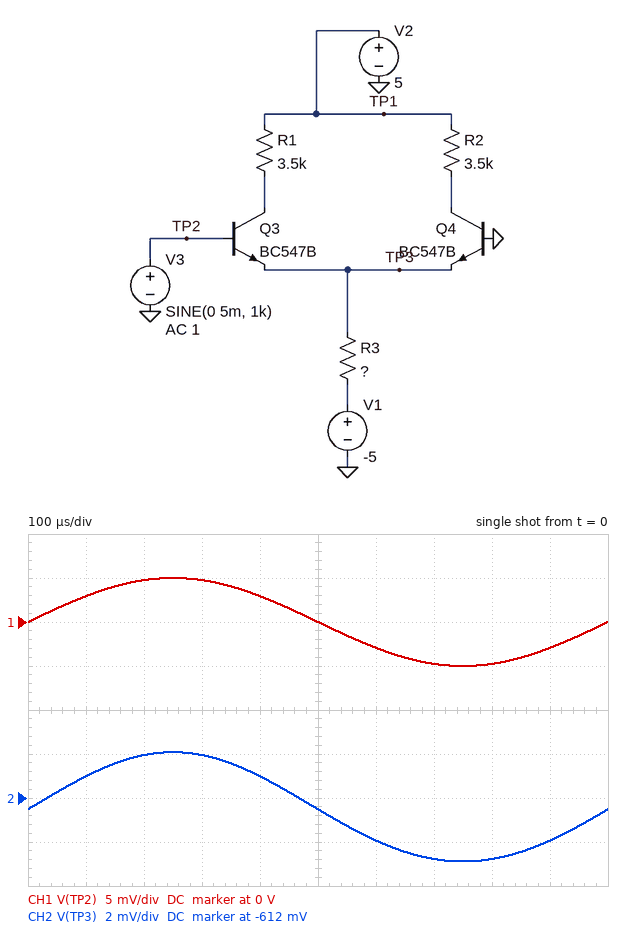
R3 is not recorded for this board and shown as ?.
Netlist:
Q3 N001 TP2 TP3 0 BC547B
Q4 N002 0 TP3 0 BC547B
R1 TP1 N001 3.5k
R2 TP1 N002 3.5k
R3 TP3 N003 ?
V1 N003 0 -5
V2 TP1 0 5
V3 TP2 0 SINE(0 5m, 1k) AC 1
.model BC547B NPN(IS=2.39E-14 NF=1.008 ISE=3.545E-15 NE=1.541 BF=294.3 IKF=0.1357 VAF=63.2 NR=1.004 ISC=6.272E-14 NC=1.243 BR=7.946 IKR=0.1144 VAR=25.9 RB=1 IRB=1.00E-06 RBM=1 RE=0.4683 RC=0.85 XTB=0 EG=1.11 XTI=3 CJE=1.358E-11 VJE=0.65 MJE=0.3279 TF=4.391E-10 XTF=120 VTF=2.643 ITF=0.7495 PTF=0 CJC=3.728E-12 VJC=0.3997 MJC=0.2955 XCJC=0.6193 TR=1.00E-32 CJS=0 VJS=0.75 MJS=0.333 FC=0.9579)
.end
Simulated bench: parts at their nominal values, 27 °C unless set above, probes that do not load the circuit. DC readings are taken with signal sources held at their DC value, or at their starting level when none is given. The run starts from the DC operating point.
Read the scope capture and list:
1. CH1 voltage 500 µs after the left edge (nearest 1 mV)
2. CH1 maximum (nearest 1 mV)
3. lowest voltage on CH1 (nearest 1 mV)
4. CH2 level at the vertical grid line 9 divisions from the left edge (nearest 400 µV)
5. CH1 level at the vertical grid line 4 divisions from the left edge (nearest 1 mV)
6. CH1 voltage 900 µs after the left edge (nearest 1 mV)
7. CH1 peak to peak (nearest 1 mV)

0 V
5 mV
-5 mV
-614.0 mV
3 mV
-3 mV
10 mV
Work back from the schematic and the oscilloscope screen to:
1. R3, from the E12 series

5.6 kΩ
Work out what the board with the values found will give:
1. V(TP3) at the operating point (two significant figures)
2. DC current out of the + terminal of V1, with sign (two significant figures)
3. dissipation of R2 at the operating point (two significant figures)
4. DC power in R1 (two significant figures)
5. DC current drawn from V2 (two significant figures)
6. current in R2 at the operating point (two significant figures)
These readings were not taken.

-610 mV
-780 µA
530 µW
530 µW
780 µA
390 µA
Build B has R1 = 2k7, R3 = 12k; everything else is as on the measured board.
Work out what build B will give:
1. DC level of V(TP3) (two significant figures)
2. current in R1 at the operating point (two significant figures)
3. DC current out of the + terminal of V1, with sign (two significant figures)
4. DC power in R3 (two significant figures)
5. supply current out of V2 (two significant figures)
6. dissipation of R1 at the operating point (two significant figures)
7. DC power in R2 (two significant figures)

-590 mV
180 µA
-370 µA
1.6 mW
370 µA
91 µW
120 µW
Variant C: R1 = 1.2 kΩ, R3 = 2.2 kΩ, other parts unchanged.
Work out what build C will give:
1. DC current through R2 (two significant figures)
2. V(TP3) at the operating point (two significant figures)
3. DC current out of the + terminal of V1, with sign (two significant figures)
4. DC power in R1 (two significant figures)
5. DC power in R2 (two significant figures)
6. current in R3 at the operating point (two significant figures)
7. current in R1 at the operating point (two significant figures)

970 µA
-640 mV
-2.0 mA
1.2 mW
3.3 mW
2.0 mA
1.0 mA
